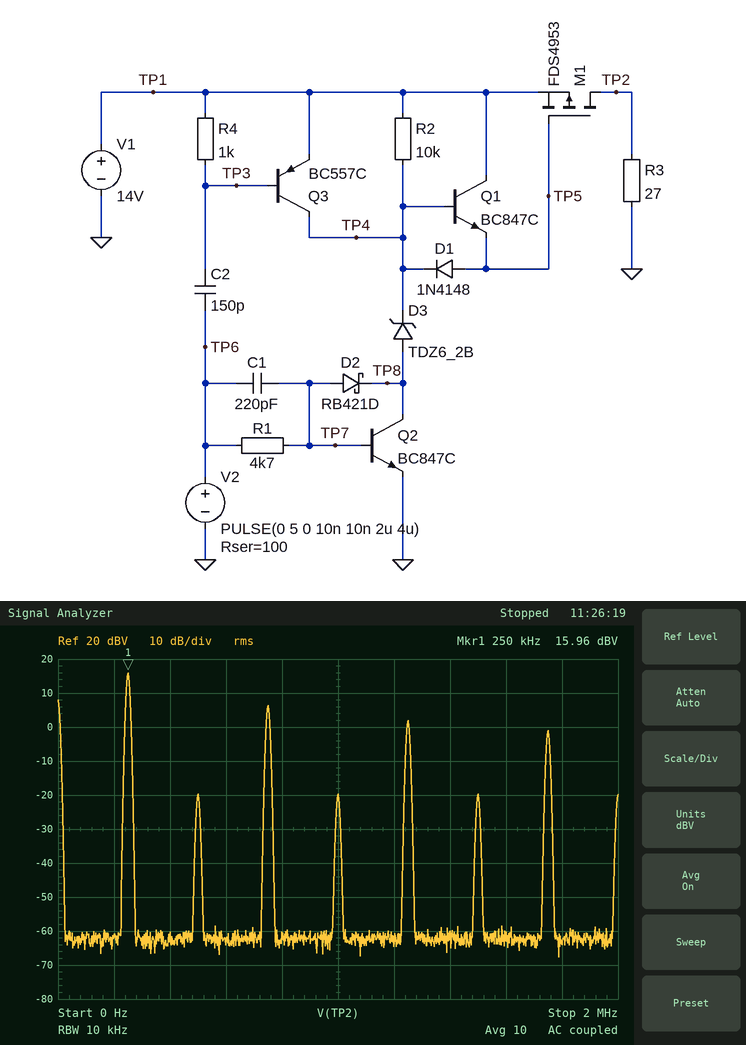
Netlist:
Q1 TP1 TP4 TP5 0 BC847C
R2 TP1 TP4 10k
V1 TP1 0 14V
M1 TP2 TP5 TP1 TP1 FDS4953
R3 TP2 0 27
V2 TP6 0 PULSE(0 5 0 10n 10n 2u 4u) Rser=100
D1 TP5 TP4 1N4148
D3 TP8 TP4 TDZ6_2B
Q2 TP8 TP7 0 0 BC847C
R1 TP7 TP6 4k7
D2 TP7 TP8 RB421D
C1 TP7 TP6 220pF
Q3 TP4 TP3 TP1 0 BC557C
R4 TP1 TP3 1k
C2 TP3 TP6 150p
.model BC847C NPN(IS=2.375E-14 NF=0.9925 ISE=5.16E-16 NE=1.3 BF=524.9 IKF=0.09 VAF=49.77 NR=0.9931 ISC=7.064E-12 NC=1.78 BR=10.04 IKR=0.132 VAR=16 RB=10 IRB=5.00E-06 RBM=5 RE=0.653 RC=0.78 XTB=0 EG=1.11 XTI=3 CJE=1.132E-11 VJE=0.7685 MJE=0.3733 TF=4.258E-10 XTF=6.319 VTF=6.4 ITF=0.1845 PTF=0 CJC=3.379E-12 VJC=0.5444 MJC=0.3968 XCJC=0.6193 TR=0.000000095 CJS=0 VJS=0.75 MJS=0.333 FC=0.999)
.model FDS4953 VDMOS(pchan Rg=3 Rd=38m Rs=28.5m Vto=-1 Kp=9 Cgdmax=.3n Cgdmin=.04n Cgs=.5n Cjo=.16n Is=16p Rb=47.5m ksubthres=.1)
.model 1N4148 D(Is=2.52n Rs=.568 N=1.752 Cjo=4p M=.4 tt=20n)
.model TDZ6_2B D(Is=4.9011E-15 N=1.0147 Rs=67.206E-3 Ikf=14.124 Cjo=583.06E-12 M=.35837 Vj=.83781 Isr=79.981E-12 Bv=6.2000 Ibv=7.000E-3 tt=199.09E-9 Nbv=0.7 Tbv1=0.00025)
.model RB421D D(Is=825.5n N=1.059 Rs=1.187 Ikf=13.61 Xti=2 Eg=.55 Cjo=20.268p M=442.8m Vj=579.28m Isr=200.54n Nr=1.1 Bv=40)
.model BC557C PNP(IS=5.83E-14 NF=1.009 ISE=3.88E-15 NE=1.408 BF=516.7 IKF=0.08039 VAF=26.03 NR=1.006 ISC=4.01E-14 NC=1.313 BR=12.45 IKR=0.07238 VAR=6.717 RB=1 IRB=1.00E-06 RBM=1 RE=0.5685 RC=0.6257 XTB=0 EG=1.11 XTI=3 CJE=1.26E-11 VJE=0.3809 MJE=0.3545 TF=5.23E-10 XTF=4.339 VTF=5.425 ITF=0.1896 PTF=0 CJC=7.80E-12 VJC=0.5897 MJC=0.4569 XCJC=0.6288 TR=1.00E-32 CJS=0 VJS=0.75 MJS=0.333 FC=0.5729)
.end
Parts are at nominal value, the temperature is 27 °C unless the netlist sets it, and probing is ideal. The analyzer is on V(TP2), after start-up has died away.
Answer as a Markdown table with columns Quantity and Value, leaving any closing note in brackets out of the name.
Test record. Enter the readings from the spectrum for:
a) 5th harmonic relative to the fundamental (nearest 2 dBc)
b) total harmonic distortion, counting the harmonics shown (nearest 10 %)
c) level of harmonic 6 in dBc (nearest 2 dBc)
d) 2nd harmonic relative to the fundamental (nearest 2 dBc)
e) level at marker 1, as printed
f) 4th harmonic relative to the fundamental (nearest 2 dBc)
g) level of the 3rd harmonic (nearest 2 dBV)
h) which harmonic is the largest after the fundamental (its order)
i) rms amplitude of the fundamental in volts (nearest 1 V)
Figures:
| Quantity | Value |
|---|---|
| 5th harmonic relative to the fundamental | -14 dBc |
| total harmonic distortion, counting the harmonics shown | 40 % |
| level of harmonic 6 in dBc | -36 dBc |
| 2nd harmonic relative to the fundamental | -36 dBc |
| level at marker 1, as printed | 15.96 dBV |
| 4th harmonic relative to the fundamental | -36 dBc |
| level of the 3rd harmonic | 6 dBV |
| which harmonic is the largest after the fundamental | 3 |
| rms amplitude of the fundamental in volts | 6 V |
